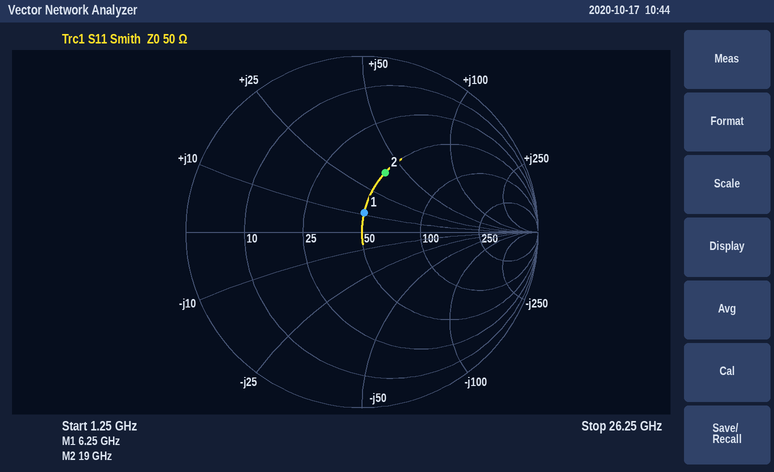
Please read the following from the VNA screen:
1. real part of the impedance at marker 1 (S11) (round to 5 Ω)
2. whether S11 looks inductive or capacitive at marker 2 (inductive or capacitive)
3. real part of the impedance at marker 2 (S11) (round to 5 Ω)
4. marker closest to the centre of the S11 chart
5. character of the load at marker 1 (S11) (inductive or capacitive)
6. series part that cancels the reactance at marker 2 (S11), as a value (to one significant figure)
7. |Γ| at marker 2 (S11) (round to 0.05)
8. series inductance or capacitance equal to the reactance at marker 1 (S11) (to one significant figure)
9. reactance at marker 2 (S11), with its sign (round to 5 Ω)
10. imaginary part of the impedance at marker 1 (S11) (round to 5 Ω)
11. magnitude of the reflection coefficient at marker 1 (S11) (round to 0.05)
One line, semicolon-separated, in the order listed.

50 Ω; inductive; 50 Ω; marker 1; inductive; 200 fF; 0.35; 300 pH; +40 Ω; +10 Ω; 0.10
